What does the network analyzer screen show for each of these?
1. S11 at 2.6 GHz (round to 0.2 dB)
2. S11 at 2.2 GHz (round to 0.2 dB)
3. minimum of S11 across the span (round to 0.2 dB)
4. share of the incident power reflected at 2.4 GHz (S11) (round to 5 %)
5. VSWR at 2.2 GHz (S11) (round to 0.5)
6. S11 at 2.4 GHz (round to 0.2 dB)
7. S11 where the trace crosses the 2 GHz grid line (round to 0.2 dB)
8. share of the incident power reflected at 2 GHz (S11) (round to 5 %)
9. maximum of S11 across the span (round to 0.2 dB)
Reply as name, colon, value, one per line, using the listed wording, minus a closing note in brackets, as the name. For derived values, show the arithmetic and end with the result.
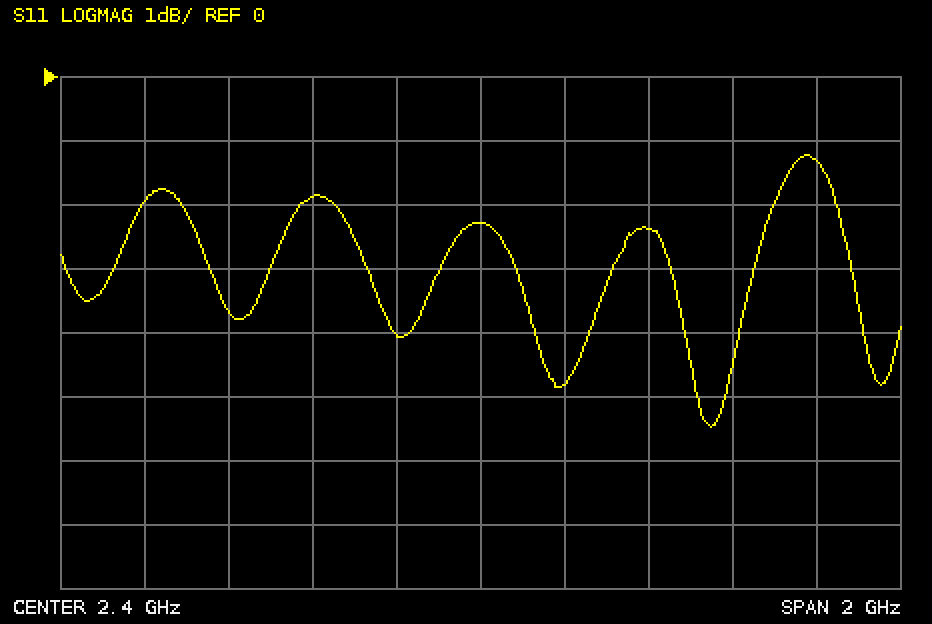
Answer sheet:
S11 at 2.6 GHz: -4.8 dB
S11 at 2.2 GHz: -4.0 dB
minimum of S11 across the span: -5.4 dB
share of the incident power reflected at 2.4 GHz (S11): 10^(-2.2/10) ≈ 60 %
VSWR at 2.2 GHz (S11): |Γ| = 10^(-4/20) = 0.6310; VSWR = (1 + 0.6310)/(1 − 0.6310) ≈ 4.42, so 4.5 to the nearest 0.5
S11 at 2.4 GHz: -2.2 dB
S11 where the trace crosses the 2 GHz grid line: -1.8 dB
share of the incident power reflected at 2 GHz (S11): 10^(-1.8/10) ≈ 66.1 %, so 65 % to the nearest 5 %
maximum of S11 across the span: -1.2 dB
